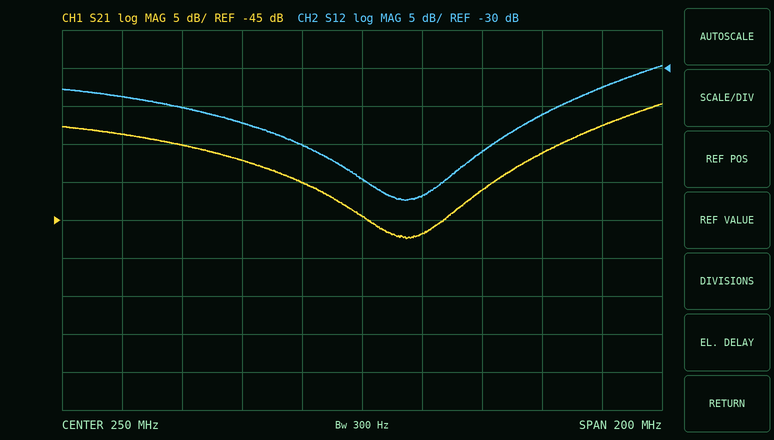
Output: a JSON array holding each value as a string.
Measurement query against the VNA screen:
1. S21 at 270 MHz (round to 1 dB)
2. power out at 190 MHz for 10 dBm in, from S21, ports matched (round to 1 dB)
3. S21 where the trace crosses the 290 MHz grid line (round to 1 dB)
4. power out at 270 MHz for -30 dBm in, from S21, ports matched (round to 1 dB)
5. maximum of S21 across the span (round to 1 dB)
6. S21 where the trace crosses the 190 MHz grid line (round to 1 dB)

["-47 dB", "-25 dBm", "-41 dB", "-77 dBm", "-30 dB", "-35 dB"]
